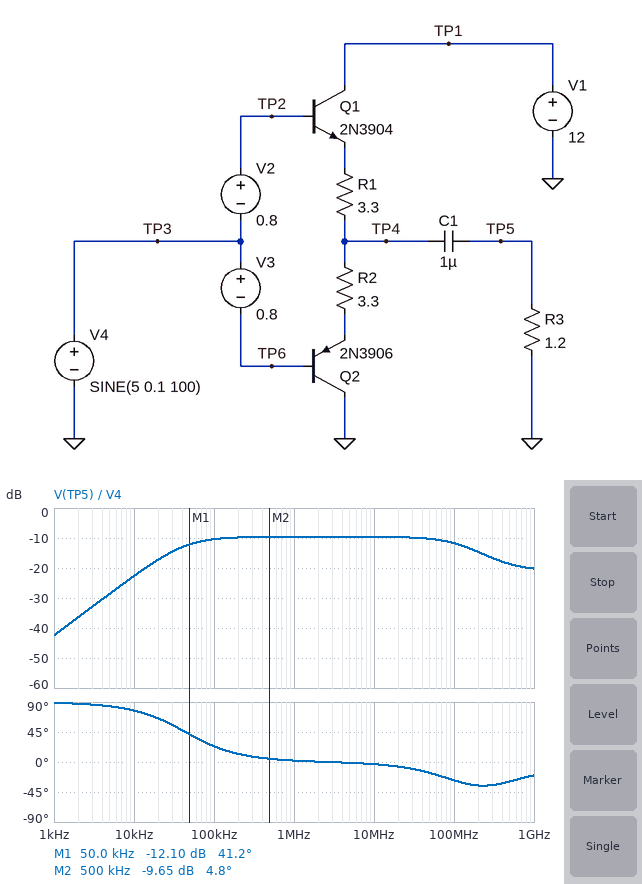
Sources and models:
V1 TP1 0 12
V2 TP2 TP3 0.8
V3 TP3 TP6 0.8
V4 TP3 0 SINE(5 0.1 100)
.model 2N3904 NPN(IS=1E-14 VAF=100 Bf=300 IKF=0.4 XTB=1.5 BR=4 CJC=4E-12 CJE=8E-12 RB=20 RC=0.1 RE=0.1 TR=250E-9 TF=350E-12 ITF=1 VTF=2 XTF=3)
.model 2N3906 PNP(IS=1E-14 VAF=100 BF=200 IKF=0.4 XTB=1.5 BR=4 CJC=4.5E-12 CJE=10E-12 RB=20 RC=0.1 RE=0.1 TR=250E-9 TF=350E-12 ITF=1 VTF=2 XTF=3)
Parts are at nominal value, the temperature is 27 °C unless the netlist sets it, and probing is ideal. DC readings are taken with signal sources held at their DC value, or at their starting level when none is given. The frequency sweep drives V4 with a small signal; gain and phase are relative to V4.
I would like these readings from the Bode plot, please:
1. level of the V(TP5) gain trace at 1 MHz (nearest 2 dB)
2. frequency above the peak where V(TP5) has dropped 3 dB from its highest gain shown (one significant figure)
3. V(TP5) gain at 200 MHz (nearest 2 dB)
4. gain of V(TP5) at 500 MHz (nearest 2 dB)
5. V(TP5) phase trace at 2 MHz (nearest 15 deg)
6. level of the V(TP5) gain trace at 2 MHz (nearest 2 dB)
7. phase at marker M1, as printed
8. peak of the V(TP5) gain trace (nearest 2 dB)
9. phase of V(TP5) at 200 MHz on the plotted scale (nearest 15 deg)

-10 dB
100 MHz
-14 dB
-18 dB
0 deg
-10 dB
41.2 deg
-10 dB
-30 deg
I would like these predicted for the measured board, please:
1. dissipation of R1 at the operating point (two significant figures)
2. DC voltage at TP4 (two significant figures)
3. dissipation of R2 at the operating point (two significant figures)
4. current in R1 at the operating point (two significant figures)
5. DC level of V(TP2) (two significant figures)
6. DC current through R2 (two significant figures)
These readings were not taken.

1.3 mW
5.0 V
1.3 mW
20 mA
5.8 V
20 mA
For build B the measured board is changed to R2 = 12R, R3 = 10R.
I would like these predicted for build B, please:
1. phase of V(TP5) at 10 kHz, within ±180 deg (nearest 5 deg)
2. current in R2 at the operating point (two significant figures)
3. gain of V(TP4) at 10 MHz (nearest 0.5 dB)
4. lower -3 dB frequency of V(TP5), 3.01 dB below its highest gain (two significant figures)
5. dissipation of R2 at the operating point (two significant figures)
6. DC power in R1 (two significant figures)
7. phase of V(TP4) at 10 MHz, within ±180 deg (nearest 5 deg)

50 deg
11 mA
-3.0 dB
11 kHz
1.4 mW
380 µW
0 deg
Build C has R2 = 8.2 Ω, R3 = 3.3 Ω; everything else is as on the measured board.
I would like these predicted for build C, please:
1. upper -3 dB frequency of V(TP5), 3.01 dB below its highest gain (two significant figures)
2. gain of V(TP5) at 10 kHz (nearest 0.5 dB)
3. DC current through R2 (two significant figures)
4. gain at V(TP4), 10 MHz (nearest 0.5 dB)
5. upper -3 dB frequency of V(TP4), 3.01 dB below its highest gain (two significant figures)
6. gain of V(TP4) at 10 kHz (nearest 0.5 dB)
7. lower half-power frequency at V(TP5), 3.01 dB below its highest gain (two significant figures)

210 MHz
-14.5 dB
13 mA
-6.5 dB
31 kHz
-0.5 dB
23 kHz
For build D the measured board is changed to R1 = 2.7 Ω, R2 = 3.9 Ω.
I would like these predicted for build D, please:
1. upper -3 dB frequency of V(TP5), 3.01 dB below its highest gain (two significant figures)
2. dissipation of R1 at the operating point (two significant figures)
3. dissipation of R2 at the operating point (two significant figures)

130 MHz
1.0 mW
1.5 mW
